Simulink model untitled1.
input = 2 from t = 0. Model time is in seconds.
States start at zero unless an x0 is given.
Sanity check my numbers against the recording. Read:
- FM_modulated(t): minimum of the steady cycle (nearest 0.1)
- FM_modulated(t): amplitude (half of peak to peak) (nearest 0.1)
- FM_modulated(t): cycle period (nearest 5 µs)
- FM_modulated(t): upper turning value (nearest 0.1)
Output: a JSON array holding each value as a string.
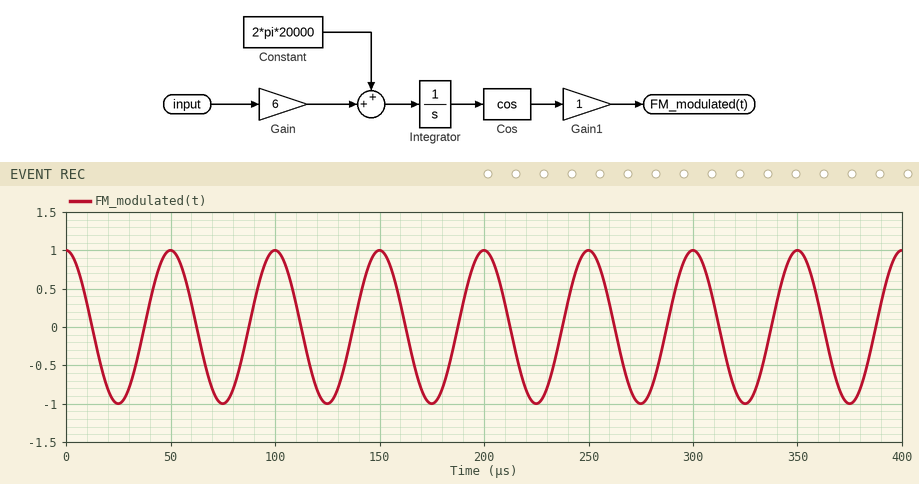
["-1.0", "1.0", "50 µs", "1.0"]
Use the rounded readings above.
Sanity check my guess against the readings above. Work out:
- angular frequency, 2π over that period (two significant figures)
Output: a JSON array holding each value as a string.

["0.13 rad/µs"]
